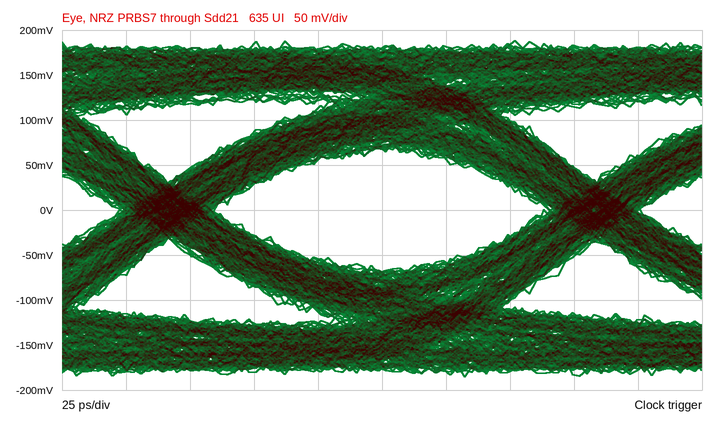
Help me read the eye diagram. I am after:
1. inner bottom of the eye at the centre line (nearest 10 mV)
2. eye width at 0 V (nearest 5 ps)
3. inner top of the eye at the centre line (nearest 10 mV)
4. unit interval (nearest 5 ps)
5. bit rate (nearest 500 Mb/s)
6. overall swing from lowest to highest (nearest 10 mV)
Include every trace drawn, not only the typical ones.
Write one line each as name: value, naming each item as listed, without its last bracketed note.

inner bottom of the eye at the centre line: -70 mV
eye width at 0 V: 130 ps
inner top of the eye at the centre line: 70 mV
unit interval: 165 ps
bit rate: 6.0 Gb/s
overall swing from lowest to highest: 370 mV
